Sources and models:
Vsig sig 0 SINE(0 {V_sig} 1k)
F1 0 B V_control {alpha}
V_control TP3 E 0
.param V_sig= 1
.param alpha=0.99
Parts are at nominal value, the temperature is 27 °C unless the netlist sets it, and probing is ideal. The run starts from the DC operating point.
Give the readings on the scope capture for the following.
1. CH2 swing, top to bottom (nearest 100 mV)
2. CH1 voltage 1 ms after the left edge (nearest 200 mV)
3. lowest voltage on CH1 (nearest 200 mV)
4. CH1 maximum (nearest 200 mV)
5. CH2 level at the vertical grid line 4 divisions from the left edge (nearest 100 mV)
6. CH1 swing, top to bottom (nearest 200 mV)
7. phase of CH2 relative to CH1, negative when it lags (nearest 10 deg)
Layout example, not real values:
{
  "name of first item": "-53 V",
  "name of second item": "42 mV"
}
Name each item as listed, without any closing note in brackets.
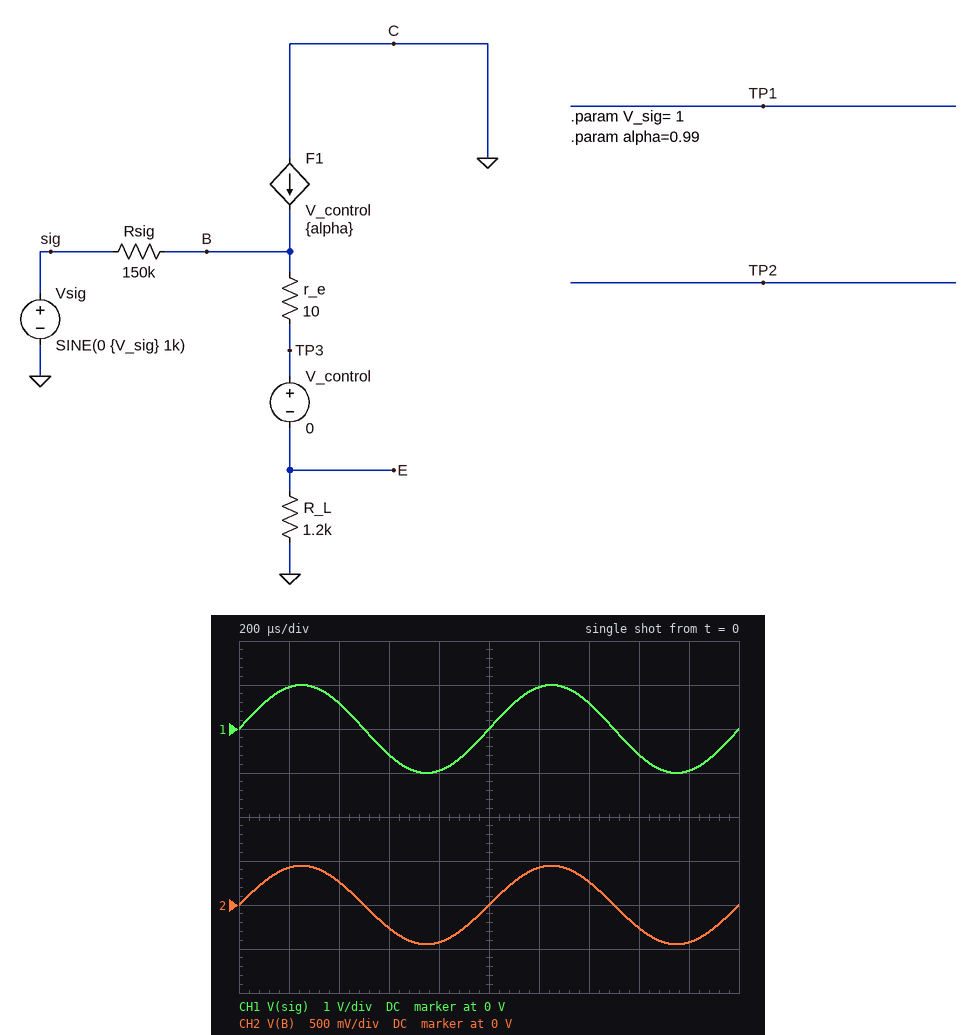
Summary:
{
  "CH2 swing, top to bottom": "900 mV",
  "CH1 voltage 1 ms after the left edge": "0 V",
  "lowest voltage on CH1": "-1.0 V",
  "CH1 maximum": "1.0 V",
  "CH2 level at the vertical grid line 4 divisions from the left edge": "-400 mV",
  "CH1 swing, top to bottom": "2.0 V",
  "phase of CH2 relative to CH1, negative when it lags": "0 deg"
}
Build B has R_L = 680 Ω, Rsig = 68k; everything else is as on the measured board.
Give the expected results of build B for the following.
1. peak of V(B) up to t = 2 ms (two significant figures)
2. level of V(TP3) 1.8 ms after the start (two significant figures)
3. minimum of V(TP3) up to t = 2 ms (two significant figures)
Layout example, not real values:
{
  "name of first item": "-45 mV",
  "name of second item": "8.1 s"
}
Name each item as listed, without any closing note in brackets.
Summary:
{
  "peak of V(B) up to t = 2 ms": "500 mV",
  "level of V(TP3) 1.8 ms after the start": "-470 mV",
  "minimum of V(TP3) up to t = 2 ms": "-500 mV"
}
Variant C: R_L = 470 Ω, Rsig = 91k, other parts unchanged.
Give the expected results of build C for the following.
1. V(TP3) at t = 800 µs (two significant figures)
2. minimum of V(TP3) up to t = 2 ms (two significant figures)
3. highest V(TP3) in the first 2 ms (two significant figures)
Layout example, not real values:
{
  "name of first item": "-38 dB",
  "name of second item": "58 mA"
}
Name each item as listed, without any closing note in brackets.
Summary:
{
  "V(TP3) at t = 800 µs": "-320 mV",
  "minimum of V(TP3) up to t = 2 ms": "-340 mV",
  "highest V(TP3) in the first 2 ms": "340 mV"
}
